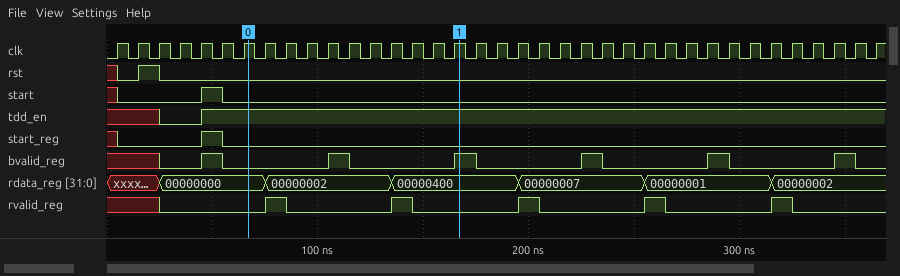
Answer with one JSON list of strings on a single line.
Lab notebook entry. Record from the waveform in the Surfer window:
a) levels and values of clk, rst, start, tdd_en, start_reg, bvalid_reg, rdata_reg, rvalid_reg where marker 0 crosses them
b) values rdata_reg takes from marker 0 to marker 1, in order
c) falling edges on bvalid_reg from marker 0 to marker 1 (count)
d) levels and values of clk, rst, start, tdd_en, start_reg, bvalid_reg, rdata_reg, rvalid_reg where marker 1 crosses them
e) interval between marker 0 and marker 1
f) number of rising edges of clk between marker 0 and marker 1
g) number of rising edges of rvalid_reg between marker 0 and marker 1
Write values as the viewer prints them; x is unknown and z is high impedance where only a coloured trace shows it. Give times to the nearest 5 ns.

["clk=1, rst=0, start=0, tdd_en=1, start_reg=0, bvalid_reg=0, rdata_reg=00000000, rvalid_reg=0", "00000000, 00000002, 00000400", "1", "clk=1, rst=0, start=0, tdd_en=1, start_reg=0, bvalid_reg=1, rdata_reg=00000400, rvalid_reg=0", "100 ns", "10", "2"]
